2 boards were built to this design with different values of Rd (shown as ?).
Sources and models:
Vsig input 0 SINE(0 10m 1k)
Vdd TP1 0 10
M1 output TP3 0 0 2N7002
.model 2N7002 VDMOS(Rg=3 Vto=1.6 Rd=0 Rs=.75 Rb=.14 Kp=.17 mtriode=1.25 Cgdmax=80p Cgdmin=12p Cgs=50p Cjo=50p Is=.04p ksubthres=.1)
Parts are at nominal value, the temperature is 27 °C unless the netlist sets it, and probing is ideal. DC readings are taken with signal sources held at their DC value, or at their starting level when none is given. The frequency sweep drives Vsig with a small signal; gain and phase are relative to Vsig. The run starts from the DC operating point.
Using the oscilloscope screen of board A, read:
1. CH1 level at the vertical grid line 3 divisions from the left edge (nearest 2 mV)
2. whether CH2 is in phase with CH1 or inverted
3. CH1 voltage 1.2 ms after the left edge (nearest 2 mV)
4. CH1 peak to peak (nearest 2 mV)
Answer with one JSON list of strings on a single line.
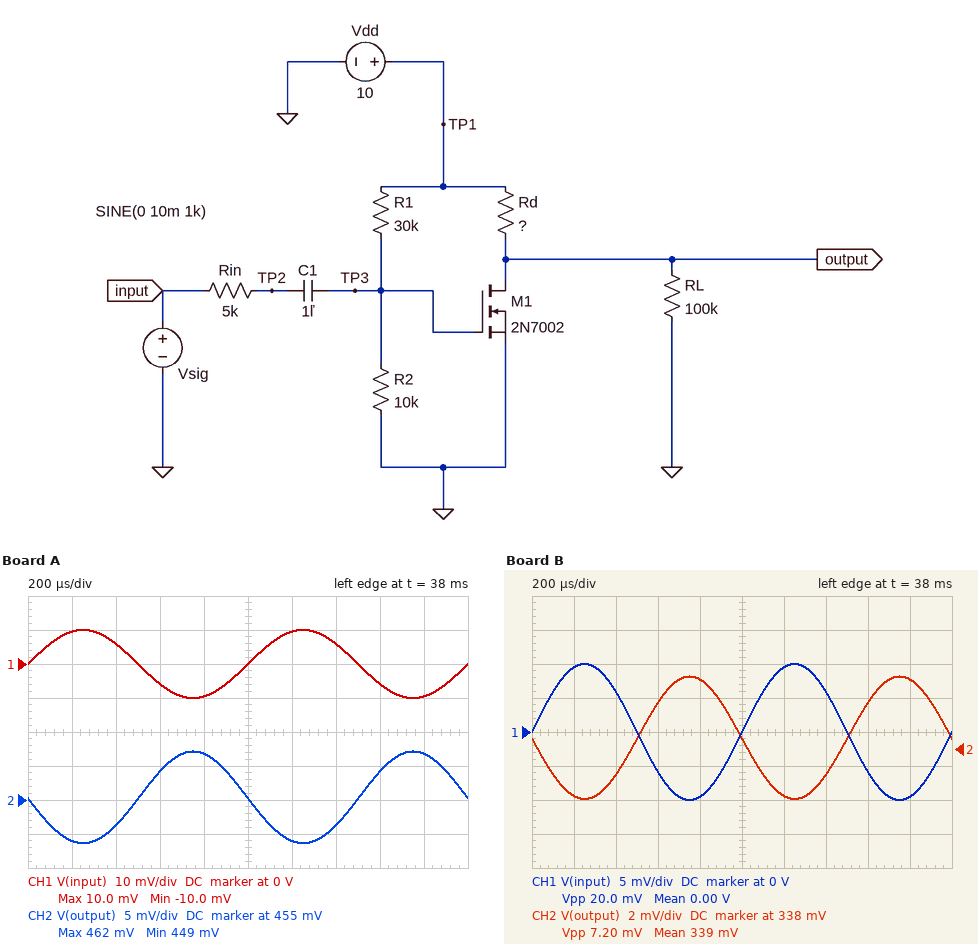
["-6 mV", "inverted", "10 mV", "20 mV"]
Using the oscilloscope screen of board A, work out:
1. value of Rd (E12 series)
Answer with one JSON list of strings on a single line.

["180 Ω"]
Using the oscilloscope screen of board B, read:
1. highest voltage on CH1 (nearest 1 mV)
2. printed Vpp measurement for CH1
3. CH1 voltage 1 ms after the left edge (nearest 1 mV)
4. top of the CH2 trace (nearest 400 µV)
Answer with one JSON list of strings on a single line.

["10 mV", "20.0 mV", "0 V", "342.4 mV"]
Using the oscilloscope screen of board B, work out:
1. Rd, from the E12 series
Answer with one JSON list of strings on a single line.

["220 Ω"]
